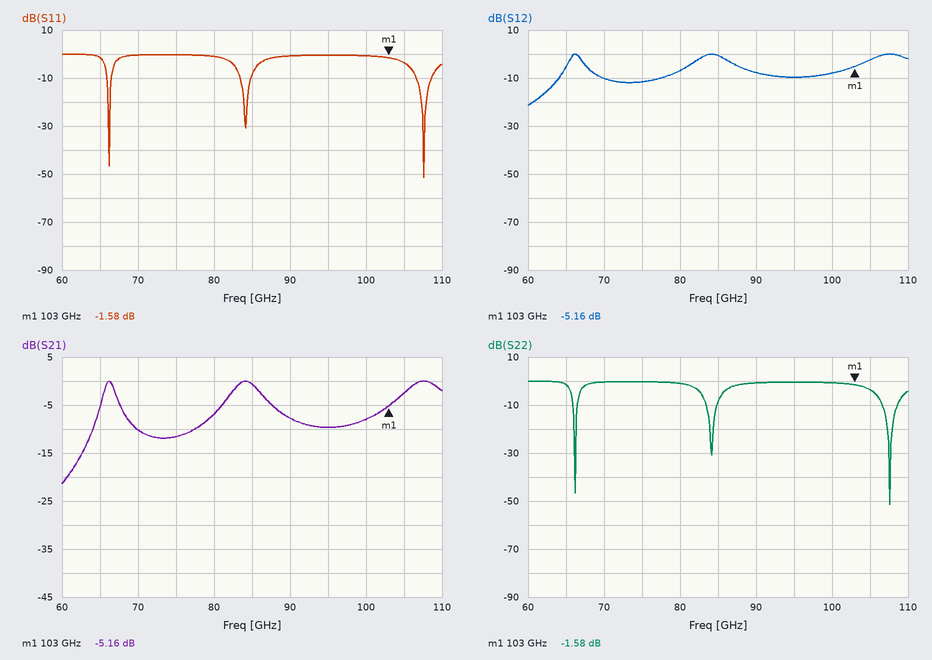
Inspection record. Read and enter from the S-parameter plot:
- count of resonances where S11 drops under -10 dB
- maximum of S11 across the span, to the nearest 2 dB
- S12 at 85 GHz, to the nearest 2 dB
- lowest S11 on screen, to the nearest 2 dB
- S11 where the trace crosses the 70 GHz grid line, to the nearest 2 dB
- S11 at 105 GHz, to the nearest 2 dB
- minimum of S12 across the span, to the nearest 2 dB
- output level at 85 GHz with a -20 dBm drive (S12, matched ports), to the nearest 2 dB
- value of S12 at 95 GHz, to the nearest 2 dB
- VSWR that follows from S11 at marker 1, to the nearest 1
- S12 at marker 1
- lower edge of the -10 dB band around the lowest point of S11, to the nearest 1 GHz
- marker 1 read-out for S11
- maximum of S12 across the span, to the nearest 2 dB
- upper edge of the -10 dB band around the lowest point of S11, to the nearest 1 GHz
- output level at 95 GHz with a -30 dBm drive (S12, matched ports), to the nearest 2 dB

3
0 dB
0 dB
-52 dB
0 dB
-4 dB
-22 dB
-20 dBm
-10 dB
11
-5.16 dB
107 GHz
-1.58 dB
0 dB
109 GHz
-40 dBm
